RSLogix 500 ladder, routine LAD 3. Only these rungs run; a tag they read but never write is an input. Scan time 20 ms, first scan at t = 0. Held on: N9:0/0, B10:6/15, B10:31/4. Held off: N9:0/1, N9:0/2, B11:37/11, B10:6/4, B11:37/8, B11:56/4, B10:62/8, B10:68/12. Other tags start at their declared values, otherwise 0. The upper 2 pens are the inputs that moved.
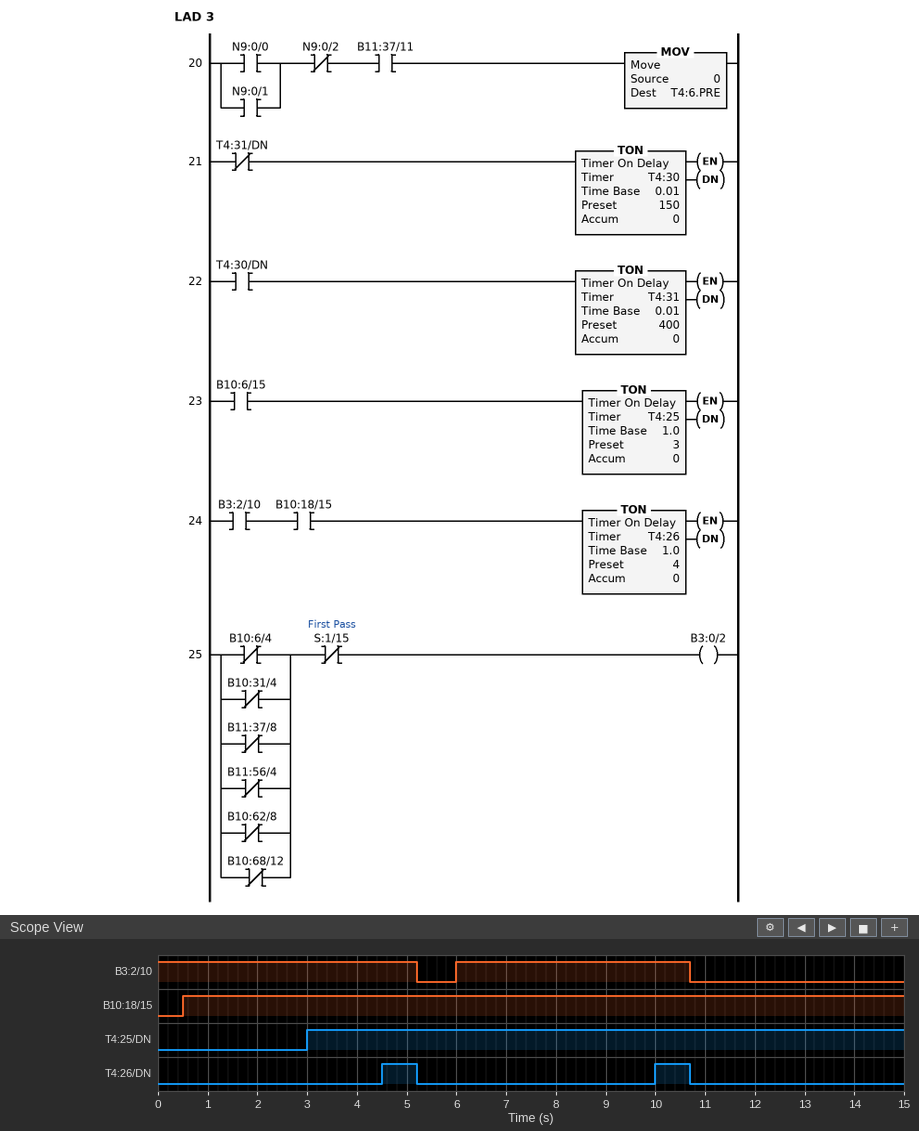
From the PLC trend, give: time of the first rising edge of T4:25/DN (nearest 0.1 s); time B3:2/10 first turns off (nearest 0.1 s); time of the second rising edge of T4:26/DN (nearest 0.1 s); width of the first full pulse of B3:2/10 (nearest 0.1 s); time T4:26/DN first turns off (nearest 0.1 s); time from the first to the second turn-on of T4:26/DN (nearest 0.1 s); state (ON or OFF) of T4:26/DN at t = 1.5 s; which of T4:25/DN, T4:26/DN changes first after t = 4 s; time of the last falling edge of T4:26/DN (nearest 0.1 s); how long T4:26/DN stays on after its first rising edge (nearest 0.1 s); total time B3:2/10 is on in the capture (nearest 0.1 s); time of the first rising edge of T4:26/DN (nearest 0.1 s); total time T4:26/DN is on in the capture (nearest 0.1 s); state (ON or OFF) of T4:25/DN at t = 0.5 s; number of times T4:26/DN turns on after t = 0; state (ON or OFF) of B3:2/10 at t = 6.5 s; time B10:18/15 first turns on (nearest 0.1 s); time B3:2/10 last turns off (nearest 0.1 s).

3.0 s
5.2 s
10.0 s
4.7 s
5.2 s
5.5 s
OFF
T4:26/DN
10.7 s
0.7 s
9.9 s
4.5 s
1.4 s
OFF
2
ON
0.5 s
10.7 s
